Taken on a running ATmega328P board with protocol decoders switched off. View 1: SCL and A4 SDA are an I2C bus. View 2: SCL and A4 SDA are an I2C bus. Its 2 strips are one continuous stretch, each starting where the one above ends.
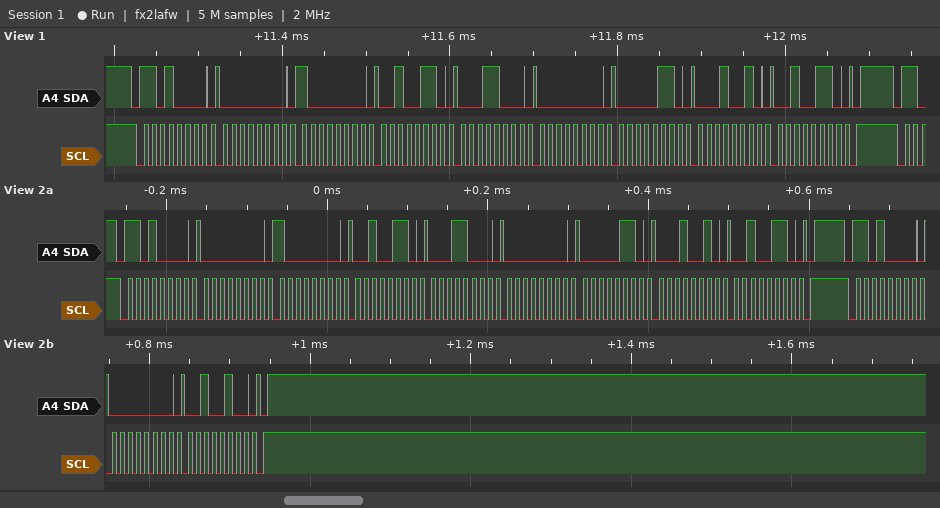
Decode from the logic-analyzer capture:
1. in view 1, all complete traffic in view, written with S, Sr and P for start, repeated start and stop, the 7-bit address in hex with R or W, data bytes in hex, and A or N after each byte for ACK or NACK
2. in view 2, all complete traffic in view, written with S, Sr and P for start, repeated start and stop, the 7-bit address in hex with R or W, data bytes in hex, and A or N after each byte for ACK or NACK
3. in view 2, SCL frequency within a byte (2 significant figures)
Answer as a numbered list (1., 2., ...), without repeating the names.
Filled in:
1. S 68W A 00 A 80 A 26 A 18 A 00 A 06 A 12 A 26 A P
2. S 68W A 00 A 80 A 26 A 18 A 00 A 06 A 12 A 26 A P S 68W A 00 A 24 A P
3. 100 kHz
